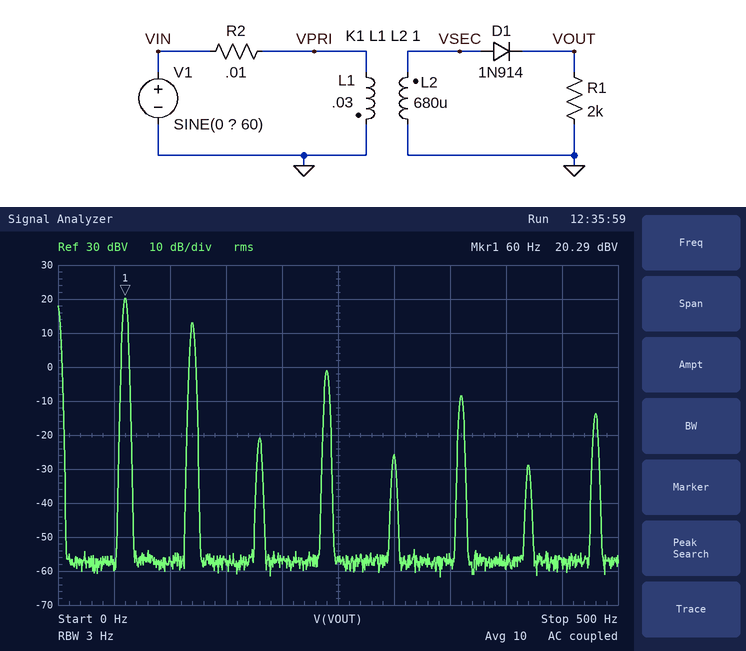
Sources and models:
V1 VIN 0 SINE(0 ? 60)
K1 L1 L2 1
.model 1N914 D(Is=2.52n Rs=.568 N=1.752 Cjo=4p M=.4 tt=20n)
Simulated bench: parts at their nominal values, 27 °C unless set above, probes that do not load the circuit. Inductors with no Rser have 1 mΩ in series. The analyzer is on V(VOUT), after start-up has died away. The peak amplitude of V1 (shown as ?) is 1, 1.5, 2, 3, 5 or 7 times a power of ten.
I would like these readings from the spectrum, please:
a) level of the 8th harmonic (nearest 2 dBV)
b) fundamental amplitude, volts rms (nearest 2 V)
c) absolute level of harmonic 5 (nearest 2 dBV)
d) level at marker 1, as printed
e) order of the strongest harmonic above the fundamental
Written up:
-14 dBV
10 V
-26 dBV
20.29 dBV
2
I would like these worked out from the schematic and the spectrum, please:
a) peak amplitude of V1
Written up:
200 V
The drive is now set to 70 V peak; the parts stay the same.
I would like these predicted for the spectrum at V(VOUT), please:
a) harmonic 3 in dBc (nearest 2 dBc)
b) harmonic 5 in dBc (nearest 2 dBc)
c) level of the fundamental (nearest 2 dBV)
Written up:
-32 dBc
-38 dBc
10 dBV
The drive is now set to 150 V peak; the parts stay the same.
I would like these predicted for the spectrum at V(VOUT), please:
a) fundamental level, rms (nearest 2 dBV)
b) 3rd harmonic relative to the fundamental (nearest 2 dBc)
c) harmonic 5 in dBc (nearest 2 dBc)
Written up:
18 dBV
-38 dBc
-44 dBc
